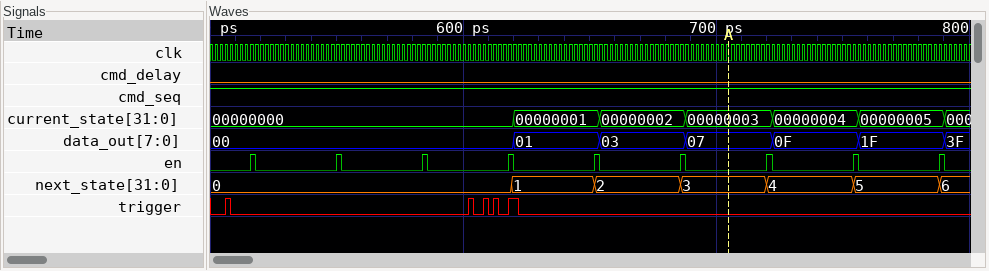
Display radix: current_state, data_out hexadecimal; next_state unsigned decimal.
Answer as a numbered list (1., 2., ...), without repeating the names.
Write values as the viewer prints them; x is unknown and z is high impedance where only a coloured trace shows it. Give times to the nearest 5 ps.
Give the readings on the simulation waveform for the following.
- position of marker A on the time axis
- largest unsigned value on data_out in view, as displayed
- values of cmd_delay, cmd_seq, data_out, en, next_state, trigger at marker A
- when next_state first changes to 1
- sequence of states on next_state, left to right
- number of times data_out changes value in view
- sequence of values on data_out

1. 705 ps
2. 3F
3. cmd_delay=0, cmd_seq=1, data_out=07, en=0, next_state=3, trigger=0
4. 620 ps
5. 0, 1, 2, 3, 4, 5, 6
6. 6
7. 00, 01, 03, 07, 0F, 1F, 3F
